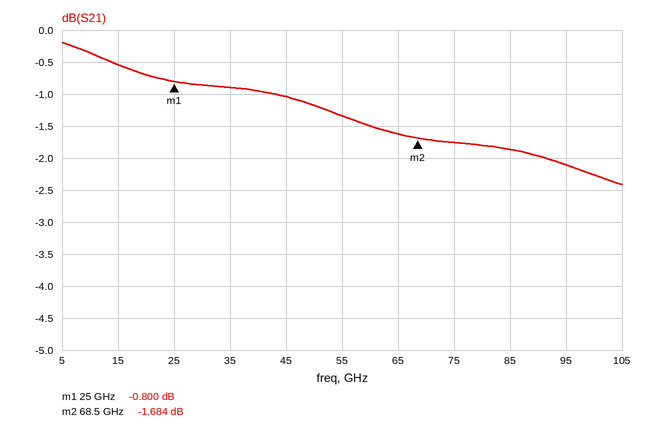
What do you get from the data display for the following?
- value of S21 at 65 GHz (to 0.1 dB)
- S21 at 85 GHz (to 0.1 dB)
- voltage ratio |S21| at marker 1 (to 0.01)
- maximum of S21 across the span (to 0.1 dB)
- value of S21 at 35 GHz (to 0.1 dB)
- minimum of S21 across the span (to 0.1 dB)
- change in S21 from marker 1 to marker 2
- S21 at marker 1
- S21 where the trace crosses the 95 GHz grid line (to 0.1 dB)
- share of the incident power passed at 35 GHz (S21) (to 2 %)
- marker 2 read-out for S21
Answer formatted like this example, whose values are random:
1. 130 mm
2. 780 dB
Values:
1. -1.6 dB
2. -1.9 dB
3. 0.91
4. -0.2 dB
5. -0.9 dB
6. -2.4 dB
7. -0.884 dB
8. -0.800 dB
9. -2.1 dB
10. 82 %
11. -1.684 dB
